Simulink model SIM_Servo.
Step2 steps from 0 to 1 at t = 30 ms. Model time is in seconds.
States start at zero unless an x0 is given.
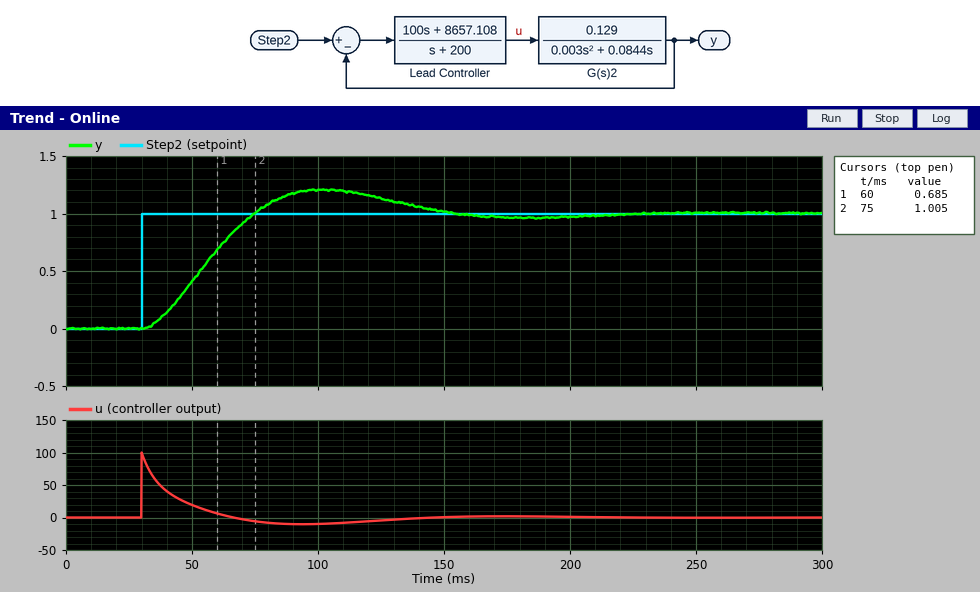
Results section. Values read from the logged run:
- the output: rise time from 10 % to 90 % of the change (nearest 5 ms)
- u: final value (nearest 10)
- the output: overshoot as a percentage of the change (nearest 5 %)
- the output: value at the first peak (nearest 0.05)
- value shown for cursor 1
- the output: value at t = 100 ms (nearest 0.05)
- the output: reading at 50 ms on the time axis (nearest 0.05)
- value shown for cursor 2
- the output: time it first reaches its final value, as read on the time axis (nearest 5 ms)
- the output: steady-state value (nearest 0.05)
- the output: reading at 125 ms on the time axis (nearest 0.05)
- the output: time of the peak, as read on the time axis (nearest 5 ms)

30 ms
0
20 %
1.20
0.685
1.20
0.40
1.005
75 ms
1.00
1.15
100 ms
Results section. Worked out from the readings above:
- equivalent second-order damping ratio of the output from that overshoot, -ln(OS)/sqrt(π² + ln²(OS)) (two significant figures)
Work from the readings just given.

0.46
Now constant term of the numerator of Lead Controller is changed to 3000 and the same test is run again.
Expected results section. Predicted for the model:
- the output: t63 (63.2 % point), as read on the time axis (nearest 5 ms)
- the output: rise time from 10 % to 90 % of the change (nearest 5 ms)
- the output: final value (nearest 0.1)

75 ms
85 ms
1.0
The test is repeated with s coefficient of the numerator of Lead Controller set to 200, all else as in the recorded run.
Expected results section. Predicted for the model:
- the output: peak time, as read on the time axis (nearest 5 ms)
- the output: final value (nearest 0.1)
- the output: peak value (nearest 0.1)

95 ms
1.0
1.1
